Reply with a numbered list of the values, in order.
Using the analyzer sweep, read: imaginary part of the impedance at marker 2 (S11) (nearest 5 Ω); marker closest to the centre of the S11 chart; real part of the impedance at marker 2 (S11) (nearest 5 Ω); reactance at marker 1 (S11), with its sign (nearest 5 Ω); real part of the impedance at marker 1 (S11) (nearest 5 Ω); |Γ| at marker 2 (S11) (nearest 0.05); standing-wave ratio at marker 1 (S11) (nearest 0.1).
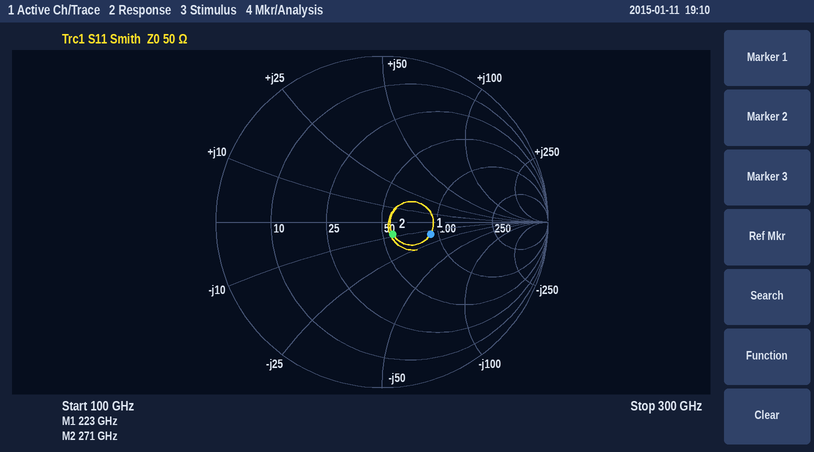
1. -10 Ω
2. marker 2
3. 55 Ω
4. -15 Ω
5. 90 Ω
6. 0.10
7. 1.9
